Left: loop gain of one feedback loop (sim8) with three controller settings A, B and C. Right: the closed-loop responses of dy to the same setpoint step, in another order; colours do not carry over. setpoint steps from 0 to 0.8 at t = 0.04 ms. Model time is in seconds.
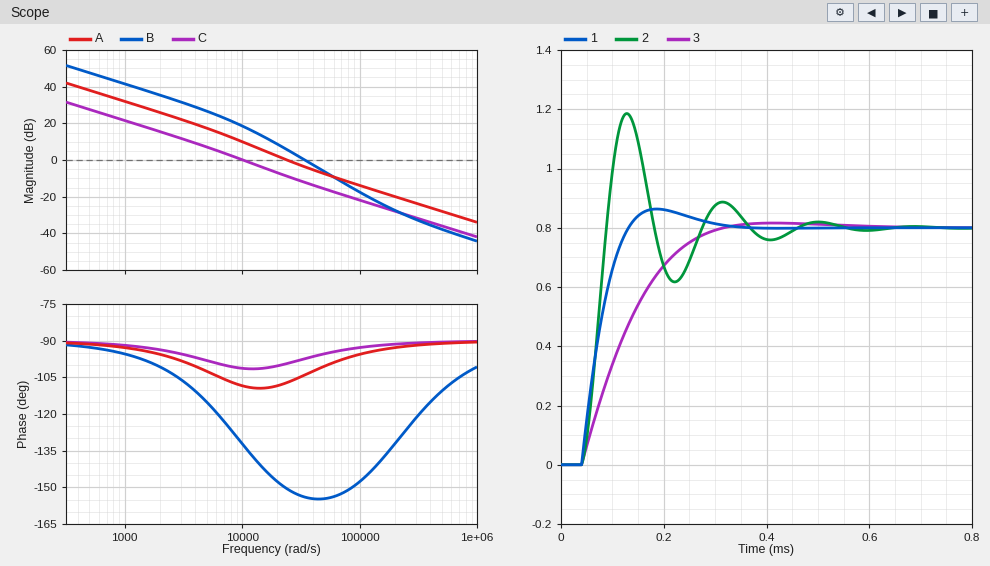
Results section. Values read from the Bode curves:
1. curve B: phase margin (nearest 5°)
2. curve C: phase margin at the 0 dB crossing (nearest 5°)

25°
80°
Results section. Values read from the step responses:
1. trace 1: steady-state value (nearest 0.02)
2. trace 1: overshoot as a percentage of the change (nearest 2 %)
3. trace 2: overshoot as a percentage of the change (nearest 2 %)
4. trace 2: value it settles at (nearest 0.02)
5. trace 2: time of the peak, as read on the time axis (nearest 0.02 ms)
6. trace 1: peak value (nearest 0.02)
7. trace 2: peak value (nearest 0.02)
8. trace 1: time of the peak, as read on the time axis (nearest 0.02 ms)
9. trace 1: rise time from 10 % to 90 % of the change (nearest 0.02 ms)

0.80
8 %
48 %
0.80
0.12 ms
0.86
1.18
0.18 ms
0.06 ms
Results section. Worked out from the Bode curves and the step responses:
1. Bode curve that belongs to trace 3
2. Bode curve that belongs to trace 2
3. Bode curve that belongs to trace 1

C
B
A
